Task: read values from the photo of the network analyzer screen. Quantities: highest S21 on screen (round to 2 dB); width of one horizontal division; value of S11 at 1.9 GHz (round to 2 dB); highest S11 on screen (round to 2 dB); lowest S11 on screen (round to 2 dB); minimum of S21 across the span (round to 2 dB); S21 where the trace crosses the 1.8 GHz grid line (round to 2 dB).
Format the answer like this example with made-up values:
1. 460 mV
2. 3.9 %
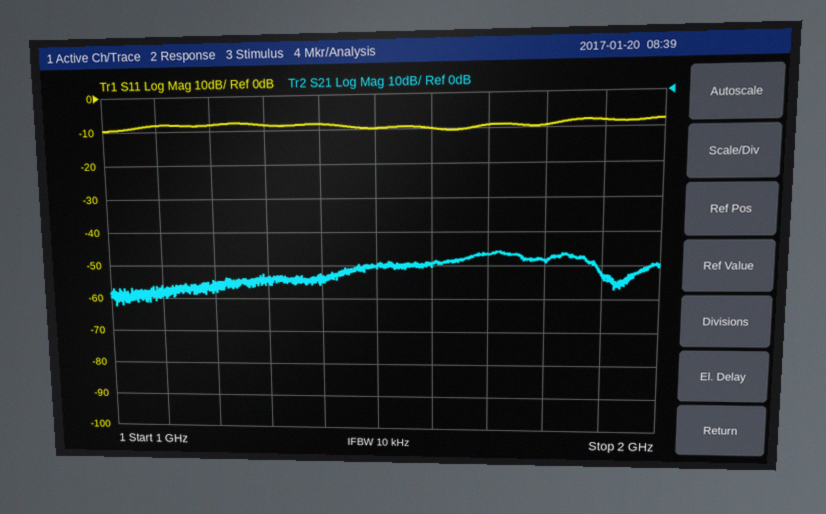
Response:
1. -46 dB
2. 100 MHz
3. -8 dB
4. -8 dB
5. -10 dB
6. -62 dB
7. -48 dB
